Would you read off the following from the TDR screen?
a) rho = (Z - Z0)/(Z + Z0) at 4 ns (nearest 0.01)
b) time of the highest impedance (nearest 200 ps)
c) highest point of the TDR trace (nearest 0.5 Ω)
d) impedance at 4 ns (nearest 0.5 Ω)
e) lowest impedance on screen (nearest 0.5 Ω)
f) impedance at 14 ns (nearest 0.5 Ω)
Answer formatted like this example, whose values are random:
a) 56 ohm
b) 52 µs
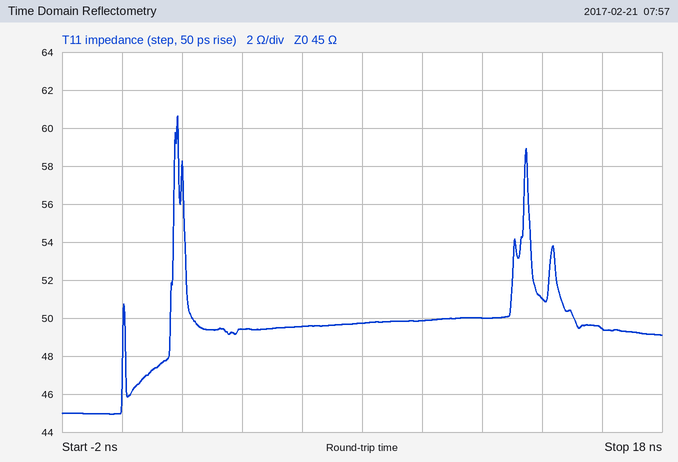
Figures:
a) +0.05
b) 1.8 ns
c) 60.5 Ω
d) 49.5 Ω
e) 45.0 Ω
f) 51.0 Ω
